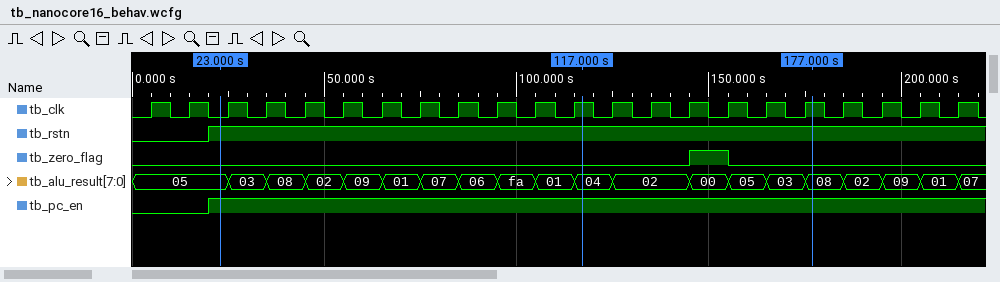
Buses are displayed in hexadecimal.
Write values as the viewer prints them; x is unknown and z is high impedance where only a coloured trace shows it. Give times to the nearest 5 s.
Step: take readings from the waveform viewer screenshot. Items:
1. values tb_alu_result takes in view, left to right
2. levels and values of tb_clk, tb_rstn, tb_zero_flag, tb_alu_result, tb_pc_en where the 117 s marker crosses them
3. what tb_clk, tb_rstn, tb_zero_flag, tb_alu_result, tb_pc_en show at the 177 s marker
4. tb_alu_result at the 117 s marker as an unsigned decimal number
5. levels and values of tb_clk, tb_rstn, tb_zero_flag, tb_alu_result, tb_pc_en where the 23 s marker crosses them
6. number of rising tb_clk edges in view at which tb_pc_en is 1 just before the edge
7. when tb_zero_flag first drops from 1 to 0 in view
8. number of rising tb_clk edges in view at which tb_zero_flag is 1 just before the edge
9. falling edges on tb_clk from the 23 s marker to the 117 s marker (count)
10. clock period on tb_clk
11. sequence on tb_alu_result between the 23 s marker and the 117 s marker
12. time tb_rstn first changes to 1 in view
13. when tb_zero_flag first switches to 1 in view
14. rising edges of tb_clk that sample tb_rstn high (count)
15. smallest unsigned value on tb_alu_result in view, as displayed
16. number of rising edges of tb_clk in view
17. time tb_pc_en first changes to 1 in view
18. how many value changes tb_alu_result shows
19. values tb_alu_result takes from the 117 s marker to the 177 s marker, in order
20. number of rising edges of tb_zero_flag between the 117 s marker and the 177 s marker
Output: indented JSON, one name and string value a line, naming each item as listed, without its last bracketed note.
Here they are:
{
  "values tb_alu_result takes in view, left to right": "05, 03, 08, 02, 09, 01, 07, 06, fa, 01, 04, 02, 00, 05, 03, 08, 02, 09, 01, 07",
  "levels and values of tb_clk, tb_rstn, tb_zero_flag, tb_alu_result, tb_pc_en where the 117 s marker crosses them": "tb_clk=1, tb_rstn=1, tb_zero_flag=0, tb_alu_result=04, tb_pc_en=1",
  "what tb_clk, tb_rstn, tb_zero_flag, tb_alu_result, tb_pc_en show at the 177 s marker": "tb_clk=1, tb_rstn=1, tb_zero_flag=0, tb_alu_result=08, tb_pc_en=1",
  "tb_alu_result at the 117 s marker as an unsigned decimal number": "4",
  "levels and values of tb_clk, tb_rstn, tb_zero_flag, tb_alu_result, tb_pc_en where the 23 s marker crosses them": "tb_clk=0, tb_rstn=1, tb_zero_flag=0, tb_alu_result=05, tb_pc_en=1",
  "number of rising tb_clk edges in view at which tb_pc_en is 1 just before the edge": "20",
  "when tb_zero_flag first drops from 1 to 0 in view": "155 s",
  "number of rising tb_clk edges in view at which tb_zero_flag is 1 just before the edge": "1",
  "falling edges on tb_clk from the 23 s marker to the 117 s marker": "9",
  "clock period on tb_clk": "10 s",
  "sequence on tb_alu_result between the 23 s marker and the 117 s marker": "05, 03, 08, 02, 09, 01, 07, 06, fa, 01, 04",
  "time tb_rstn first changes to 1 in view": "20 s",
  "when tb_zero_flag first switches to 1 in view": "145 s",
  "rising edges of tb_clk that sample tb_rstn high": "20",
  "smallest unsigned value on tb_alu_result in view, as displayed": "00",
  "number of rising edges of tb_clk in view": "22",
  "time tb_pc_en first changes to 1 in view": "20 s",
  "how many value changes tb_alu_result shows": "19",
  "values tb_alu_result takes from the 117 s marker to the 177 s marker, in order": "04, 02, 00, 05, 03, 08",
  "number of rising edges of tb_zero_flag between the 117 s marker and the 177 s marker": "1"
}
